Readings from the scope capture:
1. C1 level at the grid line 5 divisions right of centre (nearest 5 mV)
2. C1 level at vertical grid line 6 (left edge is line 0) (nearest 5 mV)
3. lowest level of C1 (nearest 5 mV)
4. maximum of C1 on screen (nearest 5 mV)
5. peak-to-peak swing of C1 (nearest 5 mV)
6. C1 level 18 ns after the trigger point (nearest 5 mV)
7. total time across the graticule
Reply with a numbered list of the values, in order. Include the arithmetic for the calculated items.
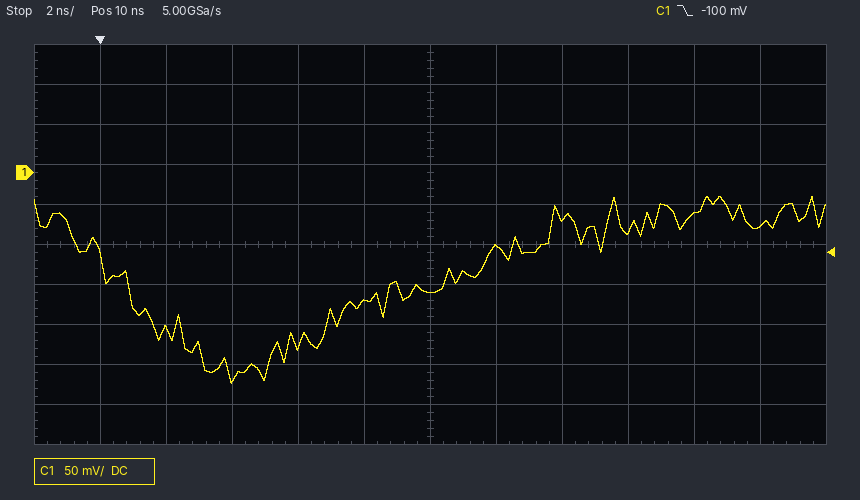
1. -65 mV
2. -150 mV
3. -265 mV
4. -30 mV
5. -30 mV − (-265 mV) = 235 mV
6. -50 mV
7. 24 ns
